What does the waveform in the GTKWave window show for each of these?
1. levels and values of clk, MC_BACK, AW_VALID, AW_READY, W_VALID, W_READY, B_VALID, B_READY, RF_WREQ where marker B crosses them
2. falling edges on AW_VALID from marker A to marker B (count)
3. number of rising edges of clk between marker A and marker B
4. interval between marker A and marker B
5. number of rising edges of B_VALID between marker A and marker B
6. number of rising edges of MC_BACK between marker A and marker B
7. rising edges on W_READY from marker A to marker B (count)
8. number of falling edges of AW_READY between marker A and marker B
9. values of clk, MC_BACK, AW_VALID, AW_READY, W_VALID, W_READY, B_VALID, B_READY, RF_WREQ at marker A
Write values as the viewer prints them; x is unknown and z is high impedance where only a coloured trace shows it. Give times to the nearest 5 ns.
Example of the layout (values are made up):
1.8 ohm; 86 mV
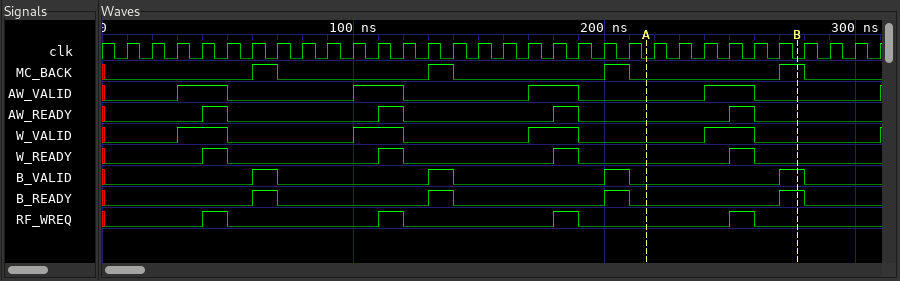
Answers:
clk=0, MC_BACK=1, AW_VALID=0, AW_READY=0, W_VALID=0, W_READY=0, B_VALID=1, B_READY=1, RF_WREQ=0; 1; 6; 60 ns; 1; 1; 1; 1; clk=0, MC_BACK=0, AW_VALID=0, AW_READY=0, W_VALID=0, W_READY=0, B_VALID=0, B_READY=0, RF_WREQ=0
